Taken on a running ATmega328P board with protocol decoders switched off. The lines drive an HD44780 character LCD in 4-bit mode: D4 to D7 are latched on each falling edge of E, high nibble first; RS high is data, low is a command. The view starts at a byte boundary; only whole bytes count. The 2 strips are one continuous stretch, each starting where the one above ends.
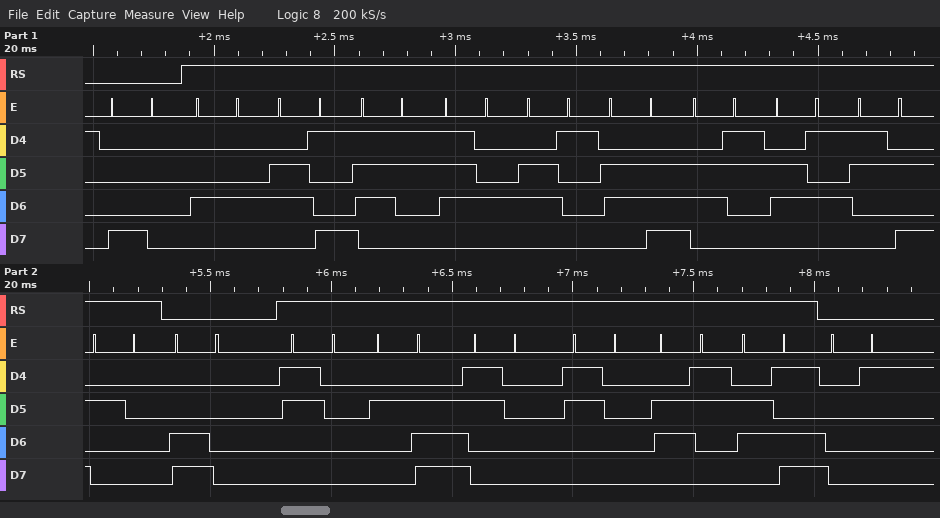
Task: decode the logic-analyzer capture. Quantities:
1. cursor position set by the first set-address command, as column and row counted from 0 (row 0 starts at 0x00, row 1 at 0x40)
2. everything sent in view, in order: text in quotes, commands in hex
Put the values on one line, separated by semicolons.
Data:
column 0, row 0; 0x80 "Distance: " 0xC0 "0.00cm" 0x01
